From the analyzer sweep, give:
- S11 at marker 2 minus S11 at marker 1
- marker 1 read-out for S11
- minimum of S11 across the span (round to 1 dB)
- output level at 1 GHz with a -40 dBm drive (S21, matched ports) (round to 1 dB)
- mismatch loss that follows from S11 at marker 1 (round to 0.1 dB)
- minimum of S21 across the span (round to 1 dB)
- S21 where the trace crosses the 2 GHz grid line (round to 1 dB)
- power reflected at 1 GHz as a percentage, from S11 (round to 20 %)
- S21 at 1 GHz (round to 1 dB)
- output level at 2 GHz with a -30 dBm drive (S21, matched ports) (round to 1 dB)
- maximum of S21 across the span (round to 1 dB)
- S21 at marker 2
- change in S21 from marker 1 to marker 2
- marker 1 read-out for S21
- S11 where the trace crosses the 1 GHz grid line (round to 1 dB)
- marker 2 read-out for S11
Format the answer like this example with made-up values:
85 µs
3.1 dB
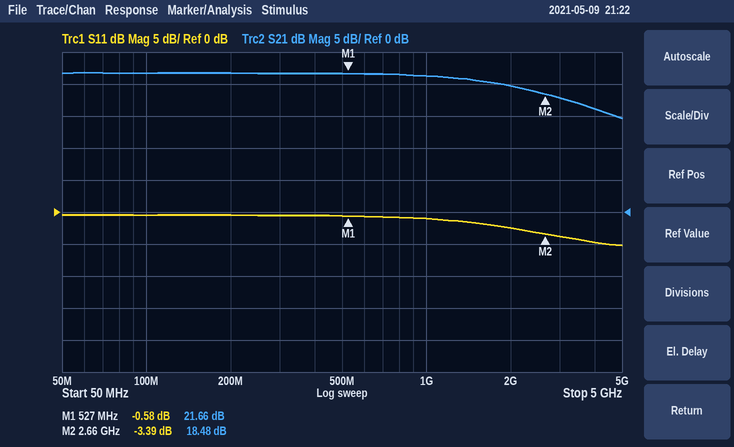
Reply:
-2.81 dB
-0.58 dB
-5 dB
-19 dBm
9.0 dB
15 dB
20 dB
80 %
21 dB
-10 dBm
22 dB
18.48 dB
-3.18 dB
21.66 dB
-1 dB
-3.39 dB
